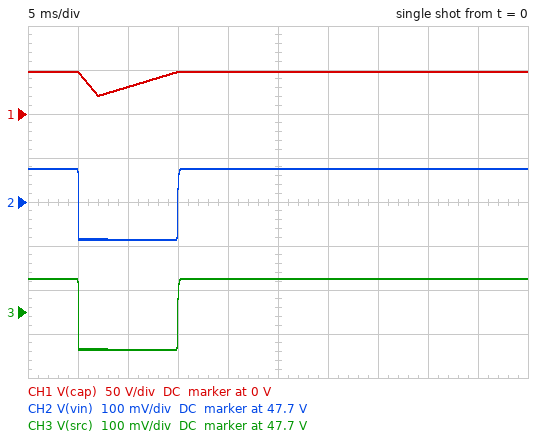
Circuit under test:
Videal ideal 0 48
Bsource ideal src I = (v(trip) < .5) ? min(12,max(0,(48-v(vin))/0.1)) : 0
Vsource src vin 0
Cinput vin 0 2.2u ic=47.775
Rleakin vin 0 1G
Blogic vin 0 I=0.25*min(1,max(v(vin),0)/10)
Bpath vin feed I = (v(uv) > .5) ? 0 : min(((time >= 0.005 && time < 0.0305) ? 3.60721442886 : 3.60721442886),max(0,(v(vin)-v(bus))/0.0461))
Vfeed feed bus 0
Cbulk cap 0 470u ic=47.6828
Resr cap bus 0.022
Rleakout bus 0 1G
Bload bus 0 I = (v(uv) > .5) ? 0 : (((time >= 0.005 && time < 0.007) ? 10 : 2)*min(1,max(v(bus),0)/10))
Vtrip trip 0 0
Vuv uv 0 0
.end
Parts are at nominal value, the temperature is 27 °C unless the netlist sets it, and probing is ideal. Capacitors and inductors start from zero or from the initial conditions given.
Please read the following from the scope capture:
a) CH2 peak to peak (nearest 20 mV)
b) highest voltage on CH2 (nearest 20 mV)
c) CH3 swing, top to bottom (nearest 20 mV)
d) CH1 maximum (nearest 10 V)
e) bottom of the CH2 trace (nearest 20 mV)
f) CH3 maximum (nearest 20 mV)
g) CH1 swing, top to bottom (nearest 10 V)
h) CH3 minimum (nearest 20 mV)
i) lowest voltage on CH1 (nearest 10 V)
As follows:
160 mV
47.78 V
160 mV
50 V
47.62 V
47.78 V
30 V
47.62 V
20 V
